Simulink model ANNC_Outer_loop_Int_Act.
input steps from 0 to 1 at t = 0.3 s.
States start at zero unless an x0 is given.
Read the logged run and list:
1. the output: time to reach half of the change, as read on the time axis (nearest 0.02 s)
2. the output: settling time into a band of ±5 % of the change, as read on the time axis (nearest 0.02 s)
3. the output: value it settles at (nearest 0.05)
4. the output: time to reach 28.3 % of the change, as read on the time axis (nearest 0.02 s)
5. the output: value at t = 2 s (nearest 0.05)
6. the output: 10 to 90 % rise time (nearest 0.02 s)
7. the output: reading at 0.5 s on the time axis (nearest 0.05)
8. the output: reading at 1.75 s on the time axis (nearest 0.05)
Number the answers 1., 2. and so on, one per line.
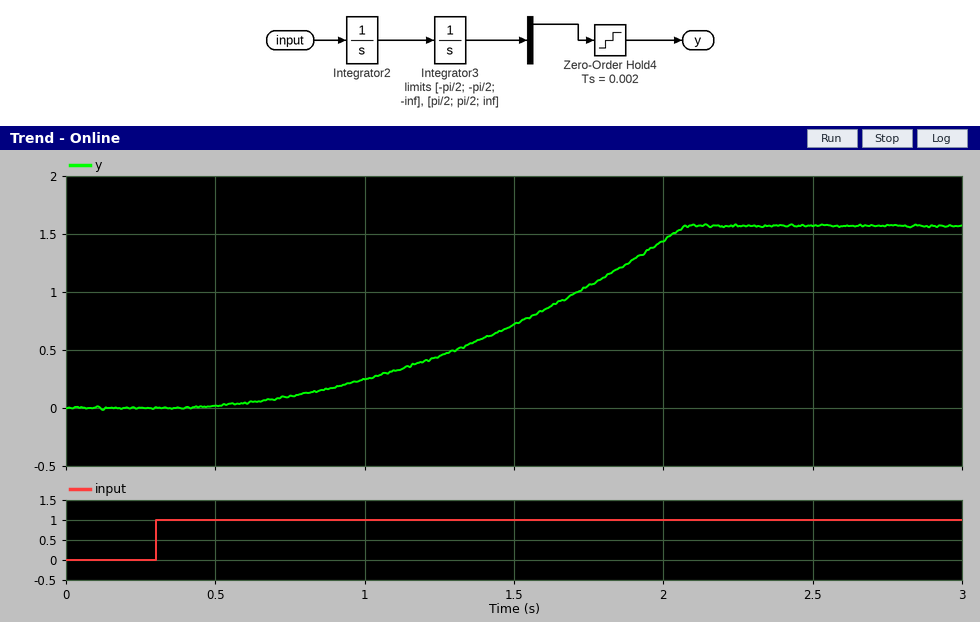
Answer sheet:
1. 1.56 s
2. 2.02 s
3. 1.55
4. 1.24 s
5. 1.45
6. 1.12 s
7. 0.00
8. 1.05
